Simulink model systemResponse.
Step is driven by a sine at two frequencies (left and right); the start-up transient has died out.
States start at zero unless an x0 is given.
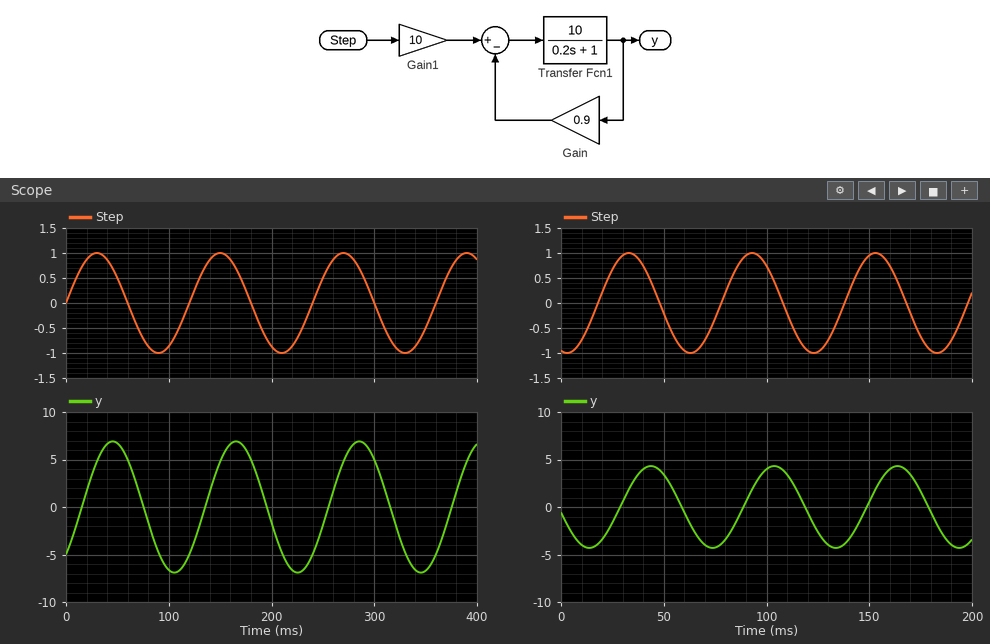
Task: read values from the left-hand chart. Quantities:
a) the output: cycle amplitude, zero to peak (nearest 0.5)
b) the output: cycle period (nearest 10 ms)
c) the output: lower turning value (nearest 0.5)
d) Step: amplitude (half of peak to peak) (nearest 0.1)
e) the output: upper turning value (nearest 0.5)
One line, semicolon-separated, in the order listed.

7.0; 120 ms; -7.0; 1.0; 7.0
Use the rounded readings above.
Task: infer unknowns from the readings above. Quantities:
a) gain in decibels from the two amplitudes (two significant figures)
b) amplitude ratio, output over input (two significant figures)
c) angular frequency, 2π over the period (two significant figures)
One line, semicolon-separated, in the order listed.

17 dB; 7.0; 0.052 rad/ms
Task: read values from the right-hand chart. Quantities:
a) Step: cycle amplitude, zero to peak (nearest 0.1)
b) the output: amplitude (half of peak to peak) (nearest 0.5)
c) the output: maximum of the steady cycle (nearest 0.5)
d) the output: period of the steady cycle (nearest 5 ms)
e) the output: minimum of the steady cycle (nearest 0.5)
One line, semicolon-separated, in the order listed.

1.0; 4.5; 4.5; 60 ms; -4.5
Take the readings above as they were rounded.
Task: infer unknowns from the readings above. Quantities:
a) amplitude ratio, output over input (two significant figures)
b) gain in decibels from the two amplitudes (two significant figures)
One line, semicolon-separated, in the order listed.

4.5; 13 dB
